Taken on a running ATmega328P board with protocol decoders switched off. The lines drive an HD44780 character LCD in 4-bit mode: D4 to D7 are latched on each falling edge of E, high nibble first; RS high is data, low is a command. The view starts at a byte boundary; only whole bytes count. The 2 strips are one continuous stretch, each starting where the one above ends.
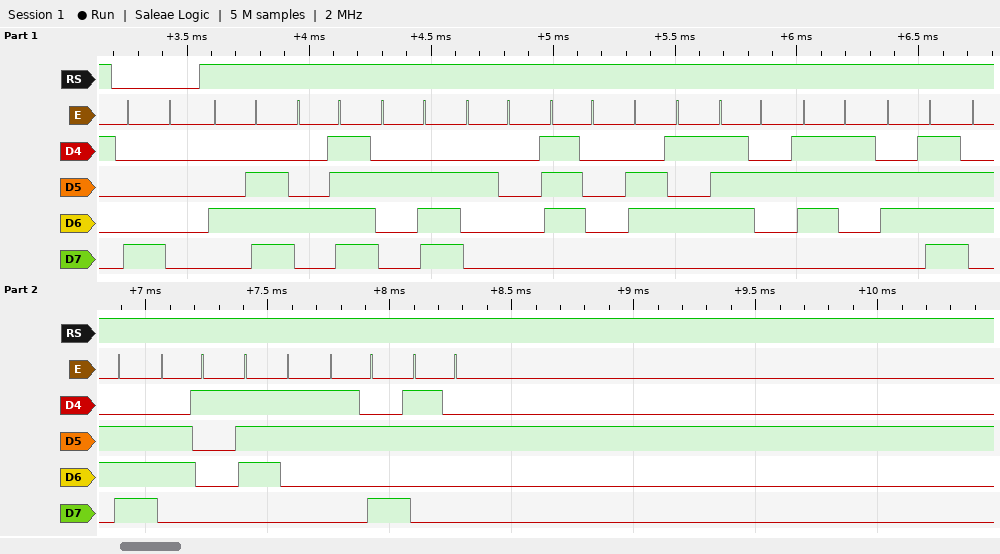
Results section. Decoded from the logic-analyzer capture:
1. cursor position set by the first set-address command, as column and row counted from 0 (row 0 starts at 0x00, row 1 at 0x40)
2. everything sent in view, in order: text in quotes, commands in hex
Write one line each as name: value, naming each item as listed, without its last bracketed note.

cursor position set by the first set-address command, as column and row counted from 0: column 0, row 0
everything sent in view, in order: text in quotes, commands in hex: 0x80 "NO. personas:2"
